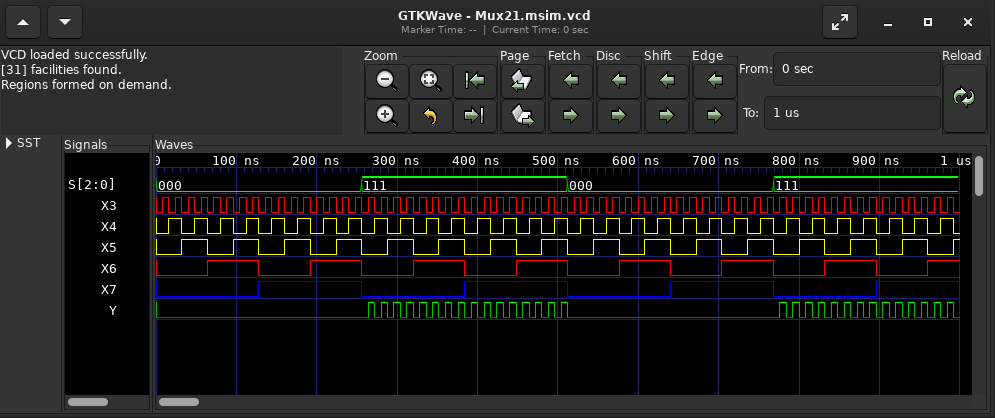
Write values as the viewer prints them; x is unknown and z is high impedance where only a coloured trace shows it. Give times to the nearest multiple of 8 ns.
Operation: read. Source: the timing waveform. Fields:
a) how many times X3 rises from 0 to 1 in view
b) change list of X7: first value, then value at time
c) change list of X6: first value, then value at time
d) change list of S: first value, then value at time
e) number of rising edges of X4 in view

62
0, 1 at 128 ns, 0 at 256 ns, 1 at 384 ns, 0 at 512 ns, 1 at 640 ns, 0 at 768 ns, 1 at 896 ns
0, 1 at 64 ns, 0 at 128 ns, 1 at 192 ns, 0 at 256 ns, 1 at 320 ns, 0 at 384 ns, 1 at 448 ns, 0 at 512 ns, 1 at 576 ns, 0 at 640 ns, 1 at 704 ns, 0 at 768 ns, 1 at 832 ns, 0 at 896 ns, 1 at 960 ns
000, 111 at 256 ns, 000 at 512 ns, 111 at 768 ns
31
